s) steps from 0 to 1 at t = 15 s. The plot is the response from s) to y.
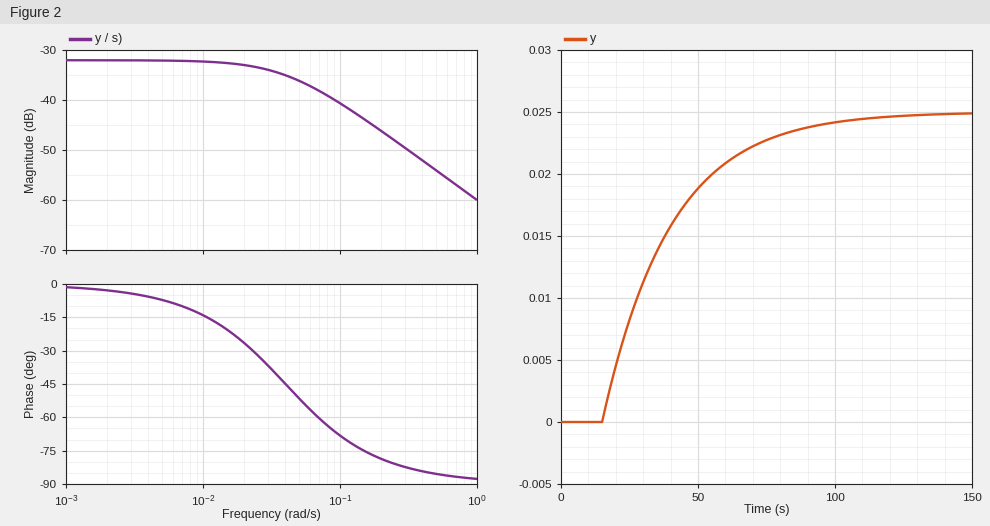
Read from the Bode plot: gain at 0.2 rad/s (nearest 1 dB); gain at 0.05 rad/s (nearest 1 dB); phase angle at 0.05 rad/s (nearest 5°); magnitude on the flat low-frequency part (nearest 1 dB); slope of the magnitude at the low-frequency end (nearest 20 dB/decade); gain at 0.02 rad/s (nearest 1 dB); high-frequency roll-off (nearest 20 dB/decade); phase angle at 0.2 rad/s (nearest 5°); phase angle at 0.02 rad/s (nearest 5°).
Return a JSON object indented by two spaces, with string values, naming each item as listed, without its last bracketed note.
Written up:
{
  "gain at 0.2 rad/s": "-46 dB",
  "gain at 0.05 rad/s": "-36 dB",
  "phase angle at 0.05 rad/s": "-50°",
  "magnitude on the flat low-frequency part": "-32 dB",
  "slope of the magnitude at the low-frequency end": "0 dB/decade",
  "gain at 0.02 rad/s": "-33 dB",
  "high-frequency roll-off": "-20 dB/decade",
  "phase angle at 0.2 rad/s": "-80°",
  "phase angle at 0.02 rad/s": "-25°"
}
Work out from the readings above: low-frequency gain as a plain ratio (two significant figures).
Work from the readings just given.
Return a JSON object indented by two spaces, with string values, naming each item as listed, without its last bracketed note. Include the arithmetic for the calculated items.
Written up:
{
  "low-frequency gain as a plain ratio": "10^(-32 / 20) = 0.025"
}
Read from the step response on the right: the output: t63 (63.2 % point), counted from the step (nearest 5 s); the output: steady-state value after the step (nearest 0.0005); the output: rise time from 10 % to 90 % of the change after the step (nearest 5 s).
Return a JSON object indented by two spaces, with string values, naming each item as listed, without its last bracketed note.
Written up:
{
  "the output: t63 (63.2 % point), counted from the step": "25 s",
  "the output: steady-state value after the step": "0.0250",
  "the output: rise time from 10 % to 90 % of the change after the step": "55 s"
}
